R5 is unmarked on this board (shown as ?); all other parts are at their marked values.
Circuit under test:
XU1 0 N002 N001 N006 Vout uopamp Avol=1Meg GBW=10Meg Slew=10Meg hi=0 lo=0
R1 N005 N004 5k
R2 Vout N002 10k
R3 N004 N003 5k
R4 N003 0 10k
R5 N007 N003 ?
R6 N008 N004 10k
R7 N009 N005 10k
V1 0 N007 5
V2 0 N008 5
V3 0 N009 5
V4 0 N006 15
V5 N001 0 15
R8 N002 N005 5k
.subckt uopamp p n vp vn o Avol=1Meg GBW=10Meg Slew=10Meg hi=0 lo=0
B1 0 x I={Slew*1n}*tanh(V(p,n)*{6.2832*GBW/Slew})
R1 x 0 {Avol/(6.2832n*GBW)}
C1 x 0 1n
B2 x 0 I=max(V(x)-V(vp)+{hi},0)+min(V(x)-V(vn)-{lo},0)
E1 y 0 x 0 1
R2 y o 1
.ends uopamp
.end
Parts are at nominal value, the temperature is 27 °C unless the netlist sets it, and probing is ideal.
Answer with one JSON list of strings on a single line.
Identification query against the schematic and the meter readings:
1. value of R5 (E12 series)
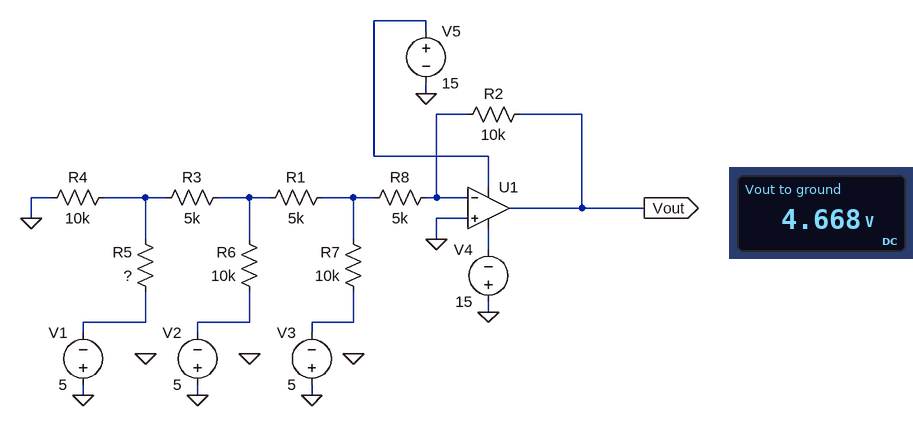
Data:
["3.9 kΩ"]
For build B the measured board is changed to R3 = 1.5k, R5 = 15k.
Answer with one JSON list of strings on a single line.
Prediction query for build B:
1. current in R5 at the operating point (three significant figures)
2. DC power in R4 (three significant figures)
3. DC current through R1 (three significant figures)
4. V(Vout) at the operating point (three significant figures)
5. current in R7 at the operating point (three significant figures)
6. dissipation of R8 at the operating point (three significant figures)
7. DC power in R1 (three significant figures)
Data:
["161 µA", "670 µW", "128 µA", "4.19 V", "291 µA", "877 µW", "82.3 µW"]
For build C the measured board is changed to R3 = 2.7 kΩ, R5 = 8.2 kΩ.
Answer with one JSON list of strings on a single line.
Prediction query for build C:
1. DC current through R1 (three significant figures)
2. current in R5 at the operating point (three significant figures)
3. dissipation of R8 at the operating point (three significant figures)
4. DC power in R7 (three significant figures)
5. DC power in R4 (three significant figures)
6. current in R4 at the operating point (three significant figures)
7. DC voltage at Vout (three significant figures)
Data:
["162 µA", "254 µA", "973 µW", "781 µW", "849 µW", "291 µA", "4.41 V"]
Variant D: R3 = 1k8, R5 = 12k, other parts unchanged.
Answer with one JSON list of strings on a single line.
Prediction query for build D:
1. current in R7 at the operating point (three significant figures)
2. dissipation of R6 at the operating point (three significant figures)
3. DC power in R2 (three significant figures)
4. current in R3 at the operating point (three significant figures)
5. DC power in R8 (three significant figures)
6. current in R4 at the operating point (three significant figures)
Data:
["287 µA", "470 µW", "1.82 mW", "77.0 µA", "910 µW", "269 µA"]
